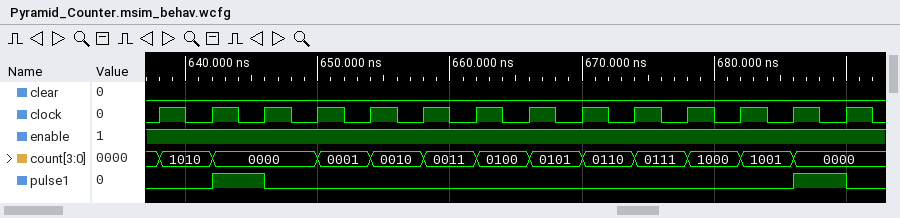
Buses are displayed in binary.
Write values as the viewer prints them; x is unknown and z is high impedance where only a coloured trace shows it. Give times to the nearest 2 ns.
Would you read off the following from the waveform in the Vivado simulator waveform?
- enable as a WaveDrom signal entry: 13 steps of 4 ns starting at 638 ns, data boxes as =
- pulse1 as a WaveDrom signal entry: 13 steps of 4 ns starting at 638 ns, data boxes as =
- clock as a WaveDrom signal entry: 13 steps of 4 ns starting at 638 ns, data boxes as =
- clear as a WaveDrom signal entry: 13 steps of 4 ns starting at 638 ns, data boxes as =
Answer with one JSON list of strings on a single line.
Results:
["{name: 'enable', wave: '1............'}", "{name: 'pulse1', wave: '010.........1'}", "{name: 'clock', wave: 'p............'}", "{name: 'clear', wave: '0............'}"]
